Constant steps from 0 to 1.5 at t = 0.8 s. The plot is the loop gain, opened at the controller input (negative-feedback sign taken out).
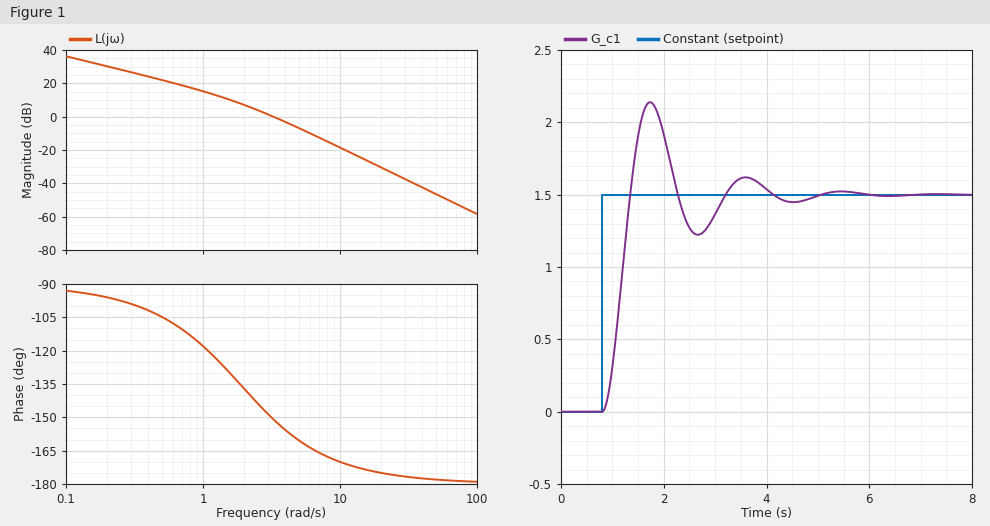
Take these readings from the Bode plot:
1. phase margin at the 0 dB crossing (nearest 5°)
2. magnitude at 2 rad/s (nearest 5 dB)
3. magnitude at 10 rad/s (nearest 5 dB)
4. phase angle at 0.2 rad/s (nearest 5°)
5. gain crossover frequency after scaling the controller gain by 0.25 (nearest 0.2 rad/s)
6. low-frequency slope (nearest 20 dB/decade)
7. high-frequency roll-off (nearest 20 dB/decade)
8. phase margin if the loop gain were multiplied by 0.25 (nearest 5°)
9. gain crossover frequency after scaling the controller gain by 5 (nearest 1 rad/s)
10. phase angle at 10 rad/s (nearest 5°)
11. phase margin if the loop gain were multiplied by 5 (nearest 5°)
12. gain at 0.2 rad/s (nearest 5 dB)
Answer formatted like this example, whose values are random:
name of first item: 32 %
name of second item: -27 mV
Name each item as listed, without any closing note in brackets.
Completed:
phase margin at the 0 dB crossing: 30°
magnitude at 2 rad/s: 5 dB
magnitude at 10 rad/s: -20 dB
phase angle at 0.2 rad/s: -95°
gain crossover frequency after scaling the controller gain by 0.25: 1.4 rad/s
low-frequency slope: -20 dB/decade
high-frequency roll-off: -40 dB/decade
phase margin if the loop gain were multiplied by 0.25: 55°
gain crossover frequency after scaling the controller gain by 5: 8 rad/s
phase angle at 10 rad/s: -170°
phase margin if the loop gain were multiplied by 5: 15°
gain at 0.2 rad/s: 30 dB
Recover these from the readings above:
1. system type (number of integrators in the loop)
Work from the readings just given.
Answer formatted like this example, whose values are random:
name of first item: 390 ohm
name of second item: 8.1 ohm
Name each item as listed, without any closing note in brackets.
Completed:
system type: 1
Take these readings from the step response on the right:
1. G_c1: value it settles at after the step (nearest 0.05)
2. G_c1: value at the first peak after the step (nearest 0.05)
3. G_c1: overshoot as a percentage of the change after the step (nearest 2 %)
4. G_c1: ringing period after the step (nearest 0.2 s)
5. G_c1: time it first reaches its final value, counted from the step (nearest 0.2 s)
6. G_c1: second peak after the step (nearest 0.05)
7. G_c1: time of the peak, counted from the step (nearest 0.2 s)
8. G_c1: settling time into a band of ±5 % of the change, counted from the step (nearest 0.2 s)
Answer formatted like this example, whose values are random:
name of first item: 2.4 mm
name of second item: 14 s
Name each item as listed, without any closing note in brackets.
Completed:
G_c1: value it settles at after the step: 1.50
G_c1: value at the first peak after the step: 2.15
G_c1: overshoot as a percentage of the change after the step: 42 %
G_c1: ringing period after the step: 1.8 s
G_c1: time it first reaches its final value, counted from the step: 0.6 s
G_c1: second peak after the step: 1.60
G_c1: time of the peak, counted from the step: 1.0 s
G_c1: settling time into a band of ±5 % of the change, counted from the step: 3.0 s
